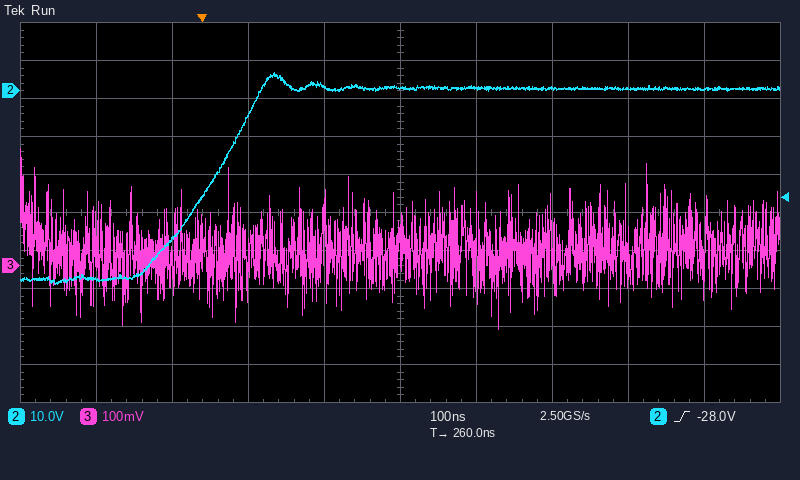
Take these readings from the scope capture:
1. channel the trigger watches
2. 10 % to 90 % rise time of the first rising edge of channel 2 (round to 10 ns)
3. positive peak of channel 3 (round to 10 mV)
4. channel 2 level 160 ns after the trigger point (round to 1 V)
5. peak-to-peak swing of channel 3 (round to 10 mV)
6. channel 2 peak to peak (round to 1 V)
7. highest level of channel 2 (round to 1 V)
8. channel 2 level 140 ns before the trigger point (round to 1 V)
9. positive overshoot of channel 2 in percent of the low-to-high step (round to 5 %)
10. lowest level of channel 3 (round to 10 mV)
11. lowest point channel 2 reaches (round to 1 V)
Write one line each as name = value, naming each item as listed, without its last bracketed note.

channel the trigger watches = channel 2
10 % to 90 % rise time of the first rising edge of channel 2 = 130 ns
positive peak of channel 3 = 310 mV
channel 2 level 160 ns after the trigger point = 1 V
peak-to-peak swing of channel 3 = 480 mV
channel 2 peak to peak = 56 V
highest level of channel 2 = 5 V
channel 2 level 140 ns before the trigger point = -50 V
positive overshoot of channel 2 in percent of the low-to-high step = 10 %
lowest level of channel 3 = -170 mV
lowest point channel 2 reaches = -51 V
